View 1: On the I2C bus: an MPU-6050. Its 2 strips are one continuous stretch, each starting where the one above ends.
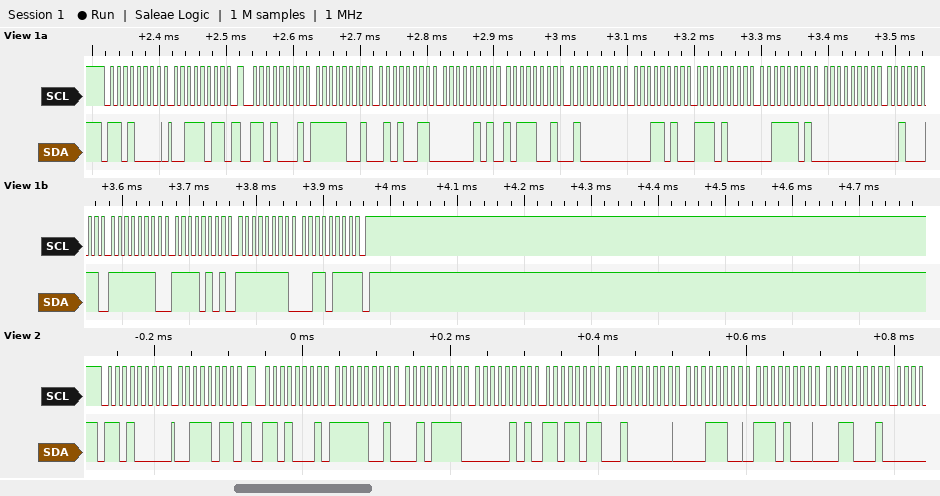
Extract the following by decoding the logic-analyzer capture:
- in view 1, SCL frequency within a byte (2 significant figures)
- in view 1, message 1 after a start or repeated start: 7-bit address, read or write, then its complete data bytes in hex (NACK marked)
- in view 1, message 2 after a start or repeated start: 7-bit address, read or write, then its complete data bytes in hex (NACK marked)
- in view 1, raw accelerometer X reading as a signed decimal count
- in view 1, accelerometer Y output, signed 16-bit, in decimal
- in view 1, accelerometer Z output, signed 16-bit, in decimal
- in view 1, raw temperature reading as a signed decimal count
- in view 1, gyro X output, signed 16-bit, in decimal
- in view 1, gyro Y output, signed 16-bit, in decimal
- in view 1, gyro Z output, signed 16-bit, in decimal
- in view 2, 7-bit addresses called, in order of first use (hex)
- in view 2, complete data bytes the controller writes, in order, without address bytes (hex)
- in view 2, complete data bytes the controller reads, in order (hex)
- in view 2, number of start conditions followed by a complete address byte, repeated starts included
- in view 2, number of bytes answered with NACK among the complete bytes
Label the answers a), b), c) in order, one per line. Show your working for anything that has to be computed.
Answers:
a) 100 kHz
b) 0x68 write: 3B
c) 0x68 read: F9 53 05 B9 40 1A E8 3D 00 23 FE F5 FF 37 NACK
d) 0xF953 = -1709
e) 0x05B9 = 1465
f) 0x401A = 16410
g) 0xE83D = -6083
h) 0x0023 = 35
i) 0xFEF5 = -267
j) 0xFF37 = -201
k) 0x68
l) 3B
m) F9 2F 05 DB 40 1C E8 31
n) 2
o) 0
